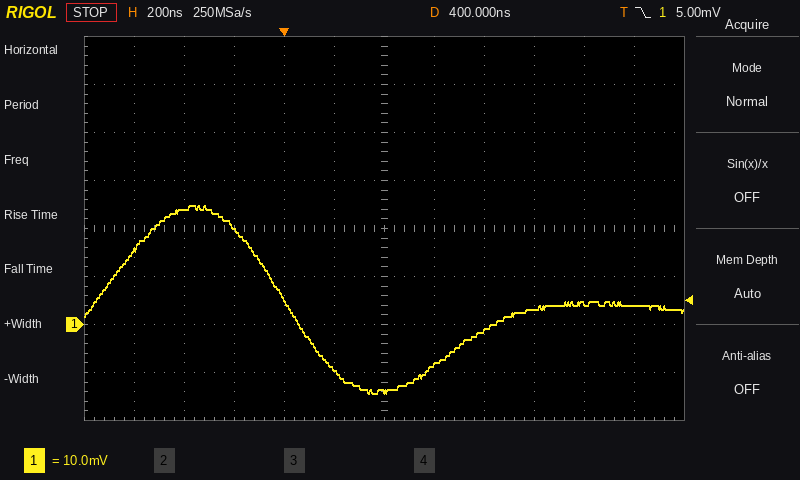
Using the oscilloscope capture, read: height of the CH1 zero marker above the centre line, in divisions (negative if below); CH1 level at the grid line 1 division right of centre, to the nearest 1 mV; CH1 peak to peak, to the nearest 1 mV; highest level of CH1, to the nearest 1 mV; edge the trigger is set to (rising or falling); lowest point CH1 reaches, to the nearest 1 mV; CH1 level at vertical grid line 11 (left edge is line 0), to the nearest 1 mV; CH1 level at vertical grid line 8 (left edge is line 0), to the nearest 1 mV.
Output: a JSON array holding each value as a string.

["-2.0 div", "-8 mV", "39 mV", "25 mV", "falling", "-14 mV", "4 mV", "-1 mV"]
